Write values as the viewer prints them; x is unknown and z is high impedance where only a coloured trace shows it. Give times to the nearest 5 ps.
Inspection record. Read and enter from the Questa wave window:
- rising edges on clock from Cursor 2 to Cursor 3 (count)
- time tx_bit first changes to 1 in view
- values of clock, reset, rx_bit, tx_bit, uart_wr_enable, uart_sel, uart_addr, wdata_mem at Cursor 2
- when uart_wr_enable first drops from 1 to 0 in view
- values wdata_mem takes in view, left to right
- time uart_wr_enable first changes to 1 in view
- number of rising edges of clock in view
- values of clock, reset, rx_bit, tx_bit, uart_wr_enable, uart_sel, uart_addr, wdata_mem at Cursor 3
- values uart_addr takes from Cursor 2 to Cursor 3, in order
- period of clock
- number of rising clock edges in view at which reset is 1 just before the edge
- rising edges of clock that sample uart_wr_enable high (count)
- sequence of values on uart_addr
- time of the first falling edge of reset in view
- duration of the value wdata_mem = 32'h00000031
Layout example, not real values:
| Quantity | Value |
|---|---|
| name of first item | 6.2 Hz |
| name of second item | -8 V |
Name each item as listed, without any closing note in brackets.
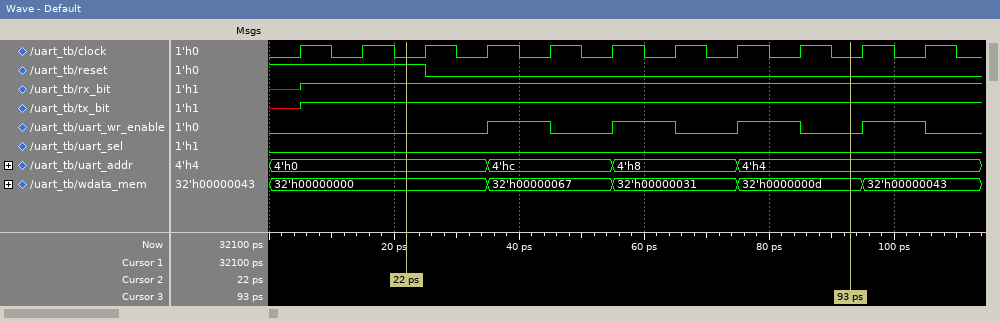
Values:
| Quantity | Value |
|---|---|
| rising edges on clock from Cursor 2 to Cursor 3 | 7 |
| time tx_bit first changes to 1 in view | 5 ps |
| values of clock, reset, rx_bit, tx_bit, uart_wr_enable, uart_sel, uart_addr, wdata_mem at Cursor 2 | clock=0, reset=1, rx_bit=1, tx_bit=1, uart_wr_enable=0, uart_sel=0, uart_addr=4'h0, wdata_mem=32'h00000000 |
| when uart_wr_enable first drops from 1 to 0 in view | 45 ps |
| values wdata_mem takes in view, left to right | 32'h00000000, 32'h00000067, 32'h00000031, 32'h0000000d, 32'h00000043 |
| time uart_wr_enable first changes to 1 in view | 35 ps |
| number of rising edges of clock in view | 11 |
| values of clock, reset, rx_bit, tx_bit, uart_wr_enable, uart_sel, uart_addr, wdata_mem at Cursor 3 | clock=0, reset=0, rx_bit=1, tx_bit=1, uart_wr_enable=0, uart_sel=0, uart_addr=4'h4, wdata_mem=32'h0000000d |
| values uart_addr takes from Cursor 2 to Cursor 3, in order | 4'h0, 4'hc, 4'h8, 4'h4 |
| period of clock | 10 ps |
| number of rising clock edges in view at which reset is 1 just before the edge | 3 |
| rising edges of clock that sample uart_wr_enable high | 4 |
| sequence of values on uart_addr | 4'h0, 4'hc, 4'h8, 4'h4 |
| time of the first falling edge of reset in view | 25 ps |
| duration of the value wdata_mem = 32'h00000031 | 20 ps |
